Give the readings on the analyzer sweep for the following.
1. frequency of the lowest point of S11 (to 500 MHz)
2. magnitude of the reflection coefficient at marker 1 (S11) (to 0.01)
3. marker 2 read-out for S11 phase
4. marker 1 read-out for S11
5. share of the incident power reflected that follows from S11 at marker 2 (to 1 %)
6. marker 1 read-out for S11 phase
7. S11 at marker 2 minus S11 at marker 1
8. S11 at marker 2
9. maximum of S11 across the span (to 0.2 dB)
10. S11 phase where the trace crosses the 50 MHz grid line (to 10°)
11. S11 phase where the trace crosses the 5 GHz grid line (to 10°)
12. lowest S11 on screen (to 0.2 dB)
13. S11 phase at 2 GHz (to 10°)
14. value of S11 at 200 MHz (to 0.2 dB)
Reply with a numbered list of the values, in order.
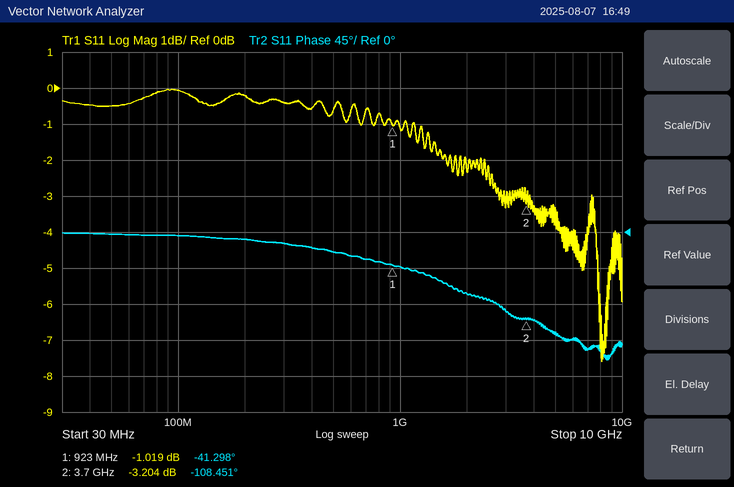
1. 8.0 GHz
2. 0.89
3. -108.451°
4. -1.019 dB
5. 48 %
6. -41.298°
7. -2.185 dB
8. -3.204 dB
9. 0.0 dB
10. 0°
11. -130°
12. -7.6 dB
13. -80°
14. -0.2 dB
